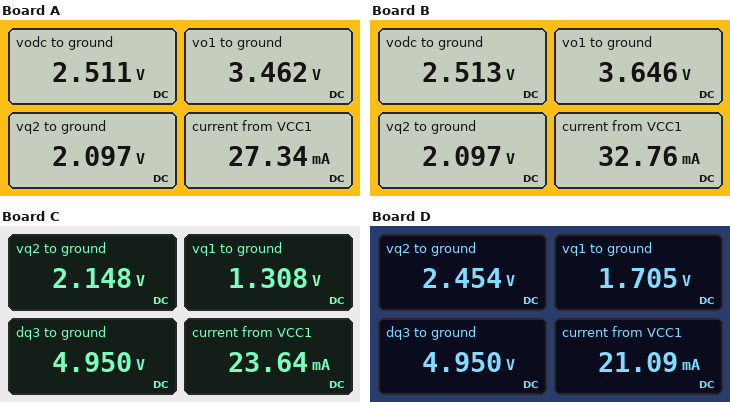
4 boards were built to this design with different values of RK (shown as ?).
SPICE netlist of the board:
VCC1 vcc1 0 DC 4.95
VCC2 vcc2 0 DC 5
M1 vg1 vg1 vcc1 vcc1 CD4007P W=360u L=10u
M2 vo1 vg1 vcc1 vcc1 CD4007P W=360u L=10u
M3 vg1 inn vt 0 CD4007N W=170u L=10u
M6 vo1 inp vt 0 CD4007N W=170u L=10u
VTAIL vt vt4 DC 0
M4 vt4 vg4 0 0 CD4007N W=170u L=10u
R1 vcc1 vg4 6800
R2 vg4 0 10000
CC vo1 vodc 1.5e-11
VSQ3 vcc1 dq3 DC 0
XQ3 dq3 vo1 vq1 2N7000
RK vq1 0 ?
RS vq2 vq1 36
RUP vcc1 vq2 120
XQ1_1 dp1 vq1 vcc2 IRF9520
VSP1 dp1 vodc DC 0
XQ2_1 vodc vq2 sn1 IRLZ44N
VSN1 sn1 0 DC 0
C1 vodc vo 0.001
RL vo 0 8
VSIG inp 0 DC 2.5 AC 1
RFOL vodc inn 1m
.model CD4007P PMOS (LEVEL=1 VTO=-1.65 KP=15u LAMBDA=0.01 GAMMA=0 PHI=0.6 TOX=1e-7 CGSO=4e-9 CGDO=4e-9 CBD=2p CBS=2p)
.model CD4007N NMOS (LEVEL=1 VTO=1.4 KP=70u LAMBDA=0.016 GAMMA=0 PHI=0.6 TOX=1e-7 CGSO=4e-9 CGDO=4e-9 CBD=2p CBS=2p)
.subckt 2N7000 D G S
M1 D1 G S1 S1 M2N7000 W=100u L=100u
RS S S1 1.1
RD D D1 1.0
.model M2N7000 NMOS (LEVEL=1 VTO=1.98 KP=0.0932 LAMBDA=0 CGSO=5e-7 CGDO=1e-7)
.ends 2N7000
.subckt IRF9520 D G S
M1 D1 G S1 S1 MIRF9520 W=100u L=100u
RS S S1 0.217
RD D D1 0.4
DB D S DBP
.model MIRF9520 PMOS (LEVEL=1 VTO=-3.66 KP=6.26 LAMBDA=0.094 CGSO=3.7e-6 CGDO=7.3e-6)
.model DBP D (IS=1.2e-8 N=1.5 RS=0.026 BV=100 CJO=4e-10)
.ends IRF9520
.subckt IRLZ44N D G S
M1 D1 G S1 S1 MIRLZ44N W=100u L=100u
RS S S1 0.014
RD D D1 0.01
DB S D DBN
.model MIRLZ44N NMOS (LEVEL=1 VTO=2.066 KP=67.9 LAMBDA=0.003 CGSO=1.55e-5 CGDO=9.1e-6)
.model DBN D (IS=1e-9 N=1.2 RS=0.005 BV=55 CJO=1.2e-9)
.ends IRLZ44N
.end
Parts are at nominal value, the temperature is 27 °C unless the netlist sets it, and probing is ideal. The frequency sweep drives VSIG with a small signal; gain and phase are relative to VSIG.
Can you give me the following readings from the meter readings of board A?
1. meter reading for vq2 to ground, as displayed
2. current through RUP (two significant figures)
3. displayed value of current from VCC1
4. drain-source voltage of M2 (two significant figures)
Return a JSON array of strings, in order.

["2.097 V", "24 mA", "27.34 mA", "-1.5 V"]
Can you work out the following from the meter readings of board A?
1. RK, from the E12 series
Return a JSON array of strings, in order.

["47 Ω"]
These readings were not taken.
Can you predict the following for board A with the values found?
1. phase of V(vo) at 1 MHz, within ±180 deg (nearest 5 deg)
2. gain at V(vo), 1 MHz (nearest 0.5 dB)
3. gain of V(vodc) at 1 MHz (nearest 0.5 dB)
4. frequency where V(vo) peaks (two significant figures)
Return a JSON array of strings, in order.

["-10 deg", "5.0 dB", "5.0 dB", "1.5 MHz"]
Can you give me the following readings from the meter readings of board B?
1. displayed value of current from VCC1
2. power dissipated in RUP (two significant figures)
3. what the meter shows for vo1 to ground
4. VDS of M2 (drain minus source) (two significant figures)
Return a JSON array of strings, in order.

["32.76 mA", "68 mW", "3.646 V", "-1.3 V"]
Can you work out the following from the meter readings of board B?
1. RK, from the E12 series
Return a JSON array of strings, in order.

["39 Ω"]
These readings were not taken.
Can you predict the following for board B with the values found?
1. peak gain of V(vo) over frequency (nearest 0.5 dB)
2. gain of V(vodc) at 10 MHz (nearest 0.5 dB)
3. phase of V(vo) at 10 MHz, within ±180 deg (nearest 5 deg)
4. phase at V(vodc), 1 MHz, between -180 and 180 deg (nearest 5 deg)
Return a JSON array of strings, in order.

["16.0 dB", "-29.0 dB", "170 deg", "-10 deg"]
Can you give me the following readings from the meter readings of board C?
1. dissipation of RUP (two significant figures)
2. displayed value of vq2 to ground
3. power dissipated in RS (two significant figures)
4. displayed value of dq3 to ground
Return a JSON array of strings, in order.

["65 mW", "2.148 V", "20 mW", "4.950 V"]
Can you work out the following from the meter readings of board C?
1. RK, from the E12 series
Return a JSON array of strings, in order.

["56 Ω"]
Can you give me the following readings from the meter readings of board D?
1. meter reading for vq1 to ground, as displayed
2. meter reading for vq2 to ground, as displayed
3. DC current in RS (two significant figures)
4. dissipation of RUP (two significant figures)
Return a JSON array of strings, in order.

["1.705 V", "2.454 V", "21 mA", "52 mW"]
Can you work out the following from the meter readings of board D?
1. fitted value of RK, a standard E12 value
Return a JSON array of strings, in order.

["82 Ω"]
